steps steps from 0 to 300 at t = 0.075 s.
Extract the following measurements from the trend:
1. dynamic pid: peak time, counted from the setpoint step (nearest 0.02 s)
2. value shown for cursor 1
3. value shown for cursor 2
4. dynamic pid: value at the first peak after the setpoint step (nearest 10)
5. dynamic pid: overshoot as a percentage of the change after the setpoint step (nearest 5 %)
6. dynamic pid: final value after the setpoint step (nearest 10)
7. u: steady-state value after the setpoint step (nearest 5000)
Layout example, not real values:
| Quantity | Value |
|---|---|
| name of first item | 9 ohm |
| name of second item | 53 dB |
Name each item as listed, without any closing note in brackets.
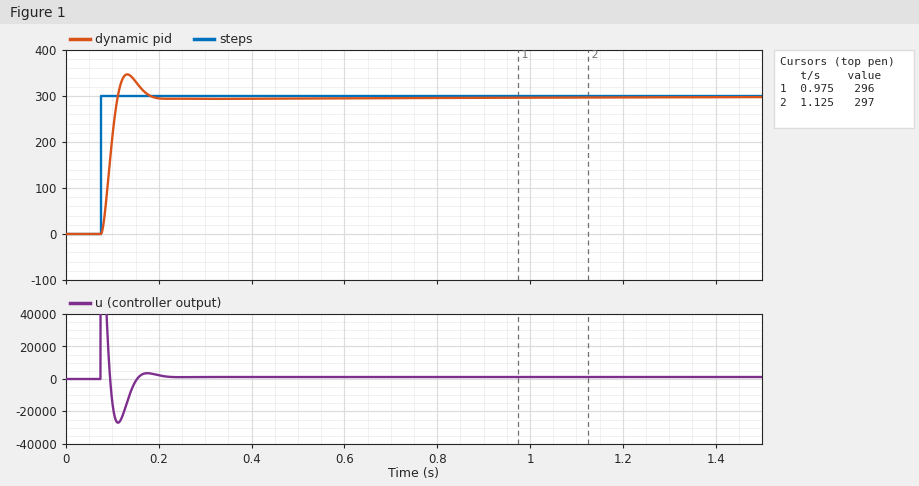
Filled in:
| Quantity | Value |
|---|---|
| dynamic pid: peak time, counted from the setpoint step | 0.06 s |
| value shown for cursor 1 | 296 |
| value shown for cursor 2 | 297 |
| dynamic pid: value at the first peak after the setpoint step | 350 |
| dynamic pid: overshoot as a percentage of the change after the setpoint step | 15 % |
| dynamic pid: final value after the setpoint step | 300 |
| u: steady-state value after the setpoint step | 0 |
